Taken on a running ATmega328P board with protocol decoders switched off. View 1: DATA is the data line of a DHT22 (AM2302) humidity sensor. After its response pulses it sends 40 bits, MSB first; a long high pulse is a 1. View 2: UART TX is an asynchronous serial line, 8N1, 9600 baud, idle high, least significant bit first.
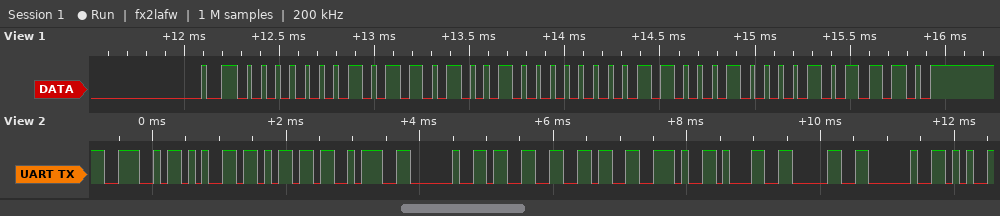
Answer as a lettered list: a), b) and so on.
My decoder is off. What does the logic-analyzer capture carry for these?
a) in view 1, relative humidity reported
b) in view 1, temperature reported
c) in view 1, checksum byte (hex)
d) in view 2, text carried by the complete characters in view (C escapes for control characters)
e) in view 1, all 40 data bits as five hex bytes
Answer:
a) 36.1 %
b) 19.6 °C
c) 0x2E
d) "Nem: 36.10 "
e) 01 69 00 C4 2E
